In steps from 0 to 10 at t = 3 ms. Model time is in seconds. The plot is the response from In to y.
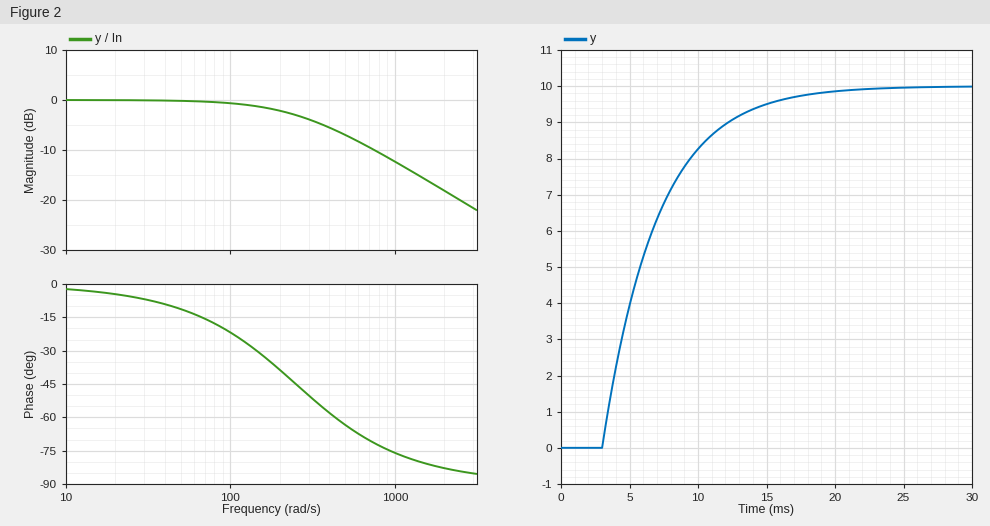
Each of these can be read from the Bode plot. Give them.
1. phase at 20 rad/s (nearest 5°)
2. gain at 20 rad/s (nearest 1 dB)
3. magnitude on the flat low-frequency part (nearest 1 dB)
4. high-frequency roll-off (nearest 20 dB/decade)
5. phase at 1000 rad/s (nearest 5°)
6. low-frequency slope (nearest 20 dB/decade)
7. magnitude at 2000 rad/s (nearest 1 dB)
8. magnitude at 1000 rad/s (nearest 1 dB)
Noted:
-5°
0 dB
0 dB
-20 dB/decade
-75°
0 dB/decade
-18 dB
-12 dB
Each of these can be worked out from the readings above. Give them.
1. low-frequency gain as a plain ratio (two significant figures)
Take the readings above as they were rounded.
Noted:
1.0
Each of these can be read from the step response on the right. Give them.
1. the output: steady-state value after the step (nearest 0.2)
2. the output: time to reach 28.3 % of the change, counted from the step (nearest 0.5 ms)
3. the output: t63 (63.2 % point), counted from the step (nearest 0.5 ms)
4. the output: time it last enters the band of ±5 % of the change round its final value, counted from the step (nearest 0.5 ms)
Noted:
10.0
1.5 ms
4.0 ms
12.0 ms
